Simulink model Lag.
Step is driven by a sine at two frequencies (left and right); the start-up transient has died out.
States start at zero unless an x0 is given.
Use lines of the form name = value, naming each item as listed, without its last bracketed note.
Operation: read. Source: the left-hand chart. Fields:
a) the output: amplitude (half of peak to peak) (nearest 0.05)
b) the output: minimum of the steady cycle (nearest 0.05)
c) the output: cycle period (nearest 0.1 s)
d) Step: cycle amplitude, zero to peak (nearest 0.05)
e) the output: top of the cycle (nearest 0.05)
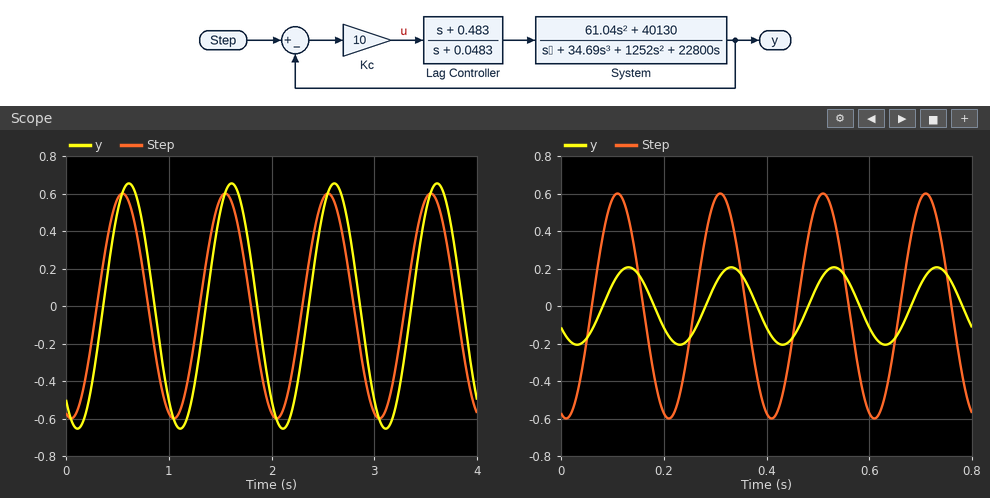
the output: amplitude (half of peak to peak) = 0.65
the output: minimum of the steady cycle = -0.65
the output: cycle period = 1.0 s
Step: cycle amplitude, zero to peak = 0.60
the output: top of the cycle = 0.65
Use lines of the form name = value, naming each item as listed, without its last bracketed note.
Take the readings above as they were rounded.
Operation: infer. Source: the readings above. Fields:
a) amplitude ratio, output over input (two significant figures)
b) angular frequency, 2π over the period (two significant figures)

amplitude ratio, output over input = 1.1
angular frequency, 2π over the period = 6.3 rad/s
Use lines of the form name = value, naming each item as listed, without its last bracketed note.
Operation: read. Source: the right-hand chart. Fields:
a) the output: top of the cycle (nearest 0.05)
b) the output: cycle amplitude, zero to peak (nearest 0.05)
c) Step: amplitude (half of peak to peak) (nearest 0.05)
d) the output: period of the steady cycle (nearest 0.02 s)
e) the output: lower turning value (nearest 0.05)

the output: top of the cycle = 0.20
the output: cycle amplitude, zero to peak = 0.20
Step: amplitude (half of peak to peak) = 0.60
the output: period of the steady cycle = 0.20 s
the output: lower turning value = -0.20
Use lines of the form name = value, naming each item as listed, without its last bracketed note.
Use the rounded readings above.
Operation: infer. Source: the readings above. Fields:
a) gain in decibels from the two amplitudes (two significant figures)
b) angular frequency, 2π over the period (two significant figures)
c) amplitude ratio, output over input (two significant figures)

gain in decibels from the two amplitudes = -9.5 dB
angular frequency, 2π over the period = 31 rad/s
amplitude ratio, output over input = 0.33
